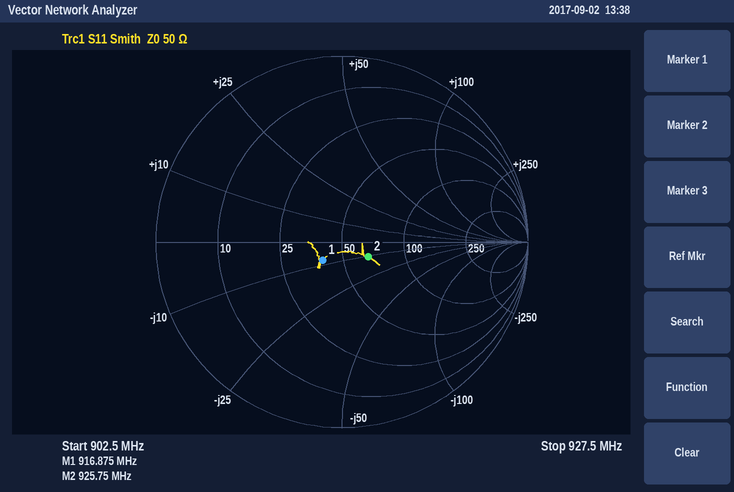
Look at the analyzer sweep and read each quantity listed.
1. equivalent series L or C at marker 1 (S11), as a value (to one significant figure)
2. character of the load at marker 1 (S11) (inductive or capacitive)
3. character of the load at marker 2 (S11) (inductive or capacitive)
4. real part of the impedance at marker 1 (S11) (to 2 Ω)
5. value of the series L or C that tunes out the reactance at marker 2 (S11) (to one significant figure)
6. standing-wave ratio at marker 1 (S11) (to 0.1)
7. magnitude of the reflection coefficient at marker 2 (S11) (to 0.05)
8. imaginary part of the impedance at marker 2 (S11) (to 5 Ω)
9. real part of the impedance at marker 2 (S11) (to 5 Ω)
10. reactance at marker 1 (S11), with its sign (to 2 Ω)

20 pF
capacitive
capacitive
40 Ω
2 nH
1.3
0.15
-10 Ω
65 Ω
-8 Ω
